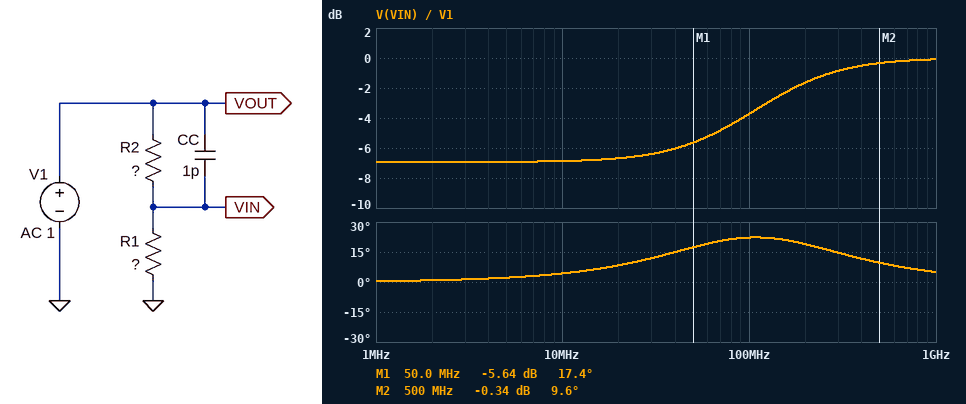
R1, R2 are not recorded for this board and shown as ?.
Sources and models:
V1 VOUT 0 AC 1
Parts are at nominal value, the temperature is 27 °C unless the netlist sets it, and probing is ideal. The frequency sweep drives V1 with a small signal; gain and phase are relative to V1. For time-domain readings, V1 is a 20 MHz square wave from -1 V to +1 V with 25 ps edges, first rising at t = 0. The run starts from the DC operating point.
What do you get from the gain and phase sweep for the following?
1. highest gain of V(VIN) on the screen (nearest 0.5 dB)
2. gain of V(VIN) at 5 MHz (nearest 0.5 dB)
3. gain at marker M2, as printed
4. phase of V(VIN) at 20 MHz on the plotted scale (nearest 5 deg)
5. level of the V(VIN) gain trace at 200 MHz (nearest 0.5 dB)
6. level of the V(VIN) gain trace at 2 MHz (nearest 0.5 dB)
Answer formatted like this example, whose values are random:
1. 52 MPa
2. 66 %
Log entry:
1. 0 dB
2. -7.0 dB
3. -0.34 dB
4. 10 deg
5. -1.5 dB
6. -7.0 dB
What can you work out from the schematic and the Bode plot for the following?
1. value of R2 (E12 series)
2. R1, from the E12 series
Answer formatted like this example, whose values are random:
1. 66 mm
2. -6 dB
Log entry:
1. 2.2 kΩ
2. 1.8 kΩ
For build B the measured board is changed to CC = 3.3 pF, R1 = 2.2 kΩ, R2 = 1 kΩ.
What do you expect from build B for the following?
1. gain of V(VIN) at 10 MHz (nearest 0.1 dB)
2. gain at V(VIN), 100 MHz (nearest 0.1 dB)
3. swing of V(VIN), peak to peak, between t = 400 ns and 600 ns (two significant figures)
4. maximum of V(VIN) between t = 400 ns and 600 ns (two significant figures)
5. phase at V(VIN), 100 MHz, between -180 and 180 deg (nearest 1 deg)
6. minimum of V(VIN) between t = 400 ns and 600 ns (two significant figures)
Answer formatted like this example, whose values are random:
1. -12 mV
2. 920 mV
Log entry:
1. -3.2 dB
2. -0.8 dB
3. 2.6 V
4. 1.3 V
5. 9 deg
6. -1.3 V
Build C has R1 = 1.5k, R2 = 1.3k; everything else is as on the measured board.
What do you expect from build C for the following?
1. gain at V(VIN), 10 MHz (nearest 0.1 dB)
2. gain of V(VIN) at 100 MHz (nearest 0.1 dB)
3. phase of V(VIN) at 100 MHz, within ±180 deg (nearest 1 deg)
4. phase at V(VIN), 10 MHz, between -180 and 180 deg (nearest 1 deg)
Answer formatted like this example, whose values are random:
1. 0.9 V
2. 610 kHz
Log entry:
1. -5.4 dB
2. -4.0 dB
3. 16 deg
4. 2 deg
